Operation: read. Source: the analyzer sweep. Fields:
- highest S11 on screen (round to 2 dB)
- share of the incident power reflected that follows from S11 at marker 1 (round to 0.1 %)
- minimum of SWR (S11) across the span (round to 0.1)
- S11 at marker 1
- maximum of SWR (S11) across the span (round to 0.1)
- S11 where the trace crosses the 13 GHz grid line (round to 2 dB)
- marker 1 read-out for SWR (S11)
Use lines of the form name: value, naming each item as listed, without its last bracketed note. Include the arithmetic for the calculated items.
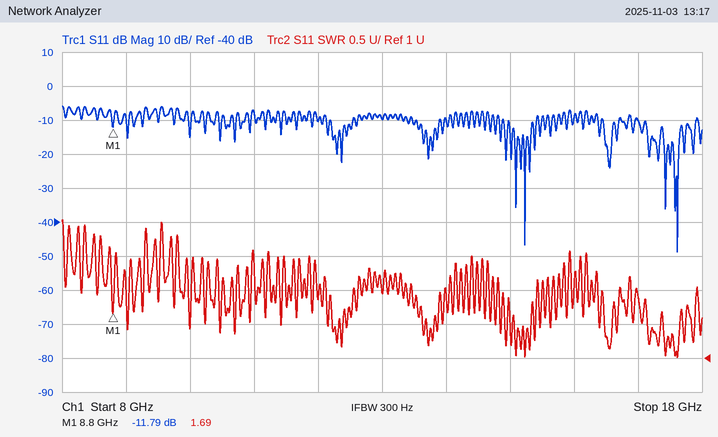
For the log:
highest S11 on screen: -6 dB
share of the incident power reflected that follows from S11 at marker 1: 10^(-11.79/10) ≈ 6.6 %
minimum of SWR (S11) across the span: 1.0
S11 at marker 1: -11.79 dB
maximum of SWR (S11) across the span: 3.0
S11 where the trace crosses the 13 GHz grid line: -10 dB
marker 1 read-out for SWR: 1.69
